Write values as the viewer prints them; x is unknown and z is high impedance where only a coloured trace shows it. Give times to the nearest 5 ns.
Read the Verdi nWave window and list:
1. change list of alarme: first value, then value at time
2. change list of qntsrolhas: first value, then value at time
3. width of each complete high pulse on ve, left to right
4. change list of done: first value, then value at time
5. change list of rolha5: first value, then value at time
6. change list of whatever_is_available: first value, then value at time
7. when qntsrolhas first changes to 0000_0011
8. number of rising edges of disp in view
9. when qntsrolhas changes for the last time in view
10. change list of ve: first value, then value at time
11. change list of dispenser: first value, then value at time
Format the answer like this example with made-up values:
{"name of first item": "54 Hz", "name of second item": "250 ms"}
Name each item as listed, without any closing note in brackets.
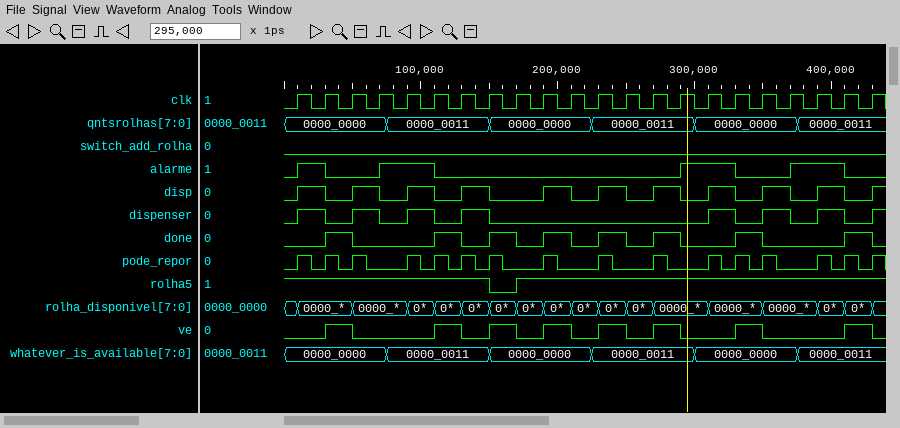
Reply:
{"change list of alarme: first value, then value at time": "0, 1 at 10 ns, 0 at 30 ns, 1 at 70 ns, 0 at 110 ns, 1 at 290 ns, 0 at 330 ns, 1 at 370 ns, 0 at 410 ns", "change list of qntsrolhas: first value, then value at time": "0000_0000, 0000_0011 at 75 ns, 0000_0000 at 150 ns, 0000_0011 at 225 ns, 0000_0000 at 300 ns, 0000_0011 at 375 ns", "width of each complete high pulse on ve, left to right": "20 ns, 20 ns, 20 ns, 20 ns, 20 ns, 20 ns, 20 ns, 20 ns", "change list of done: first value, then value at time": "0, 1 at 30 ns, 0 at 50 ns, 1 at 110 ns, 0 at 130 ns, 1 at 150 ns, 0 at 170 ns, 1 at 190 ns, 0 at 210 ns, 1 at 230 ns, 0 at 250 ns, 1 at 270 ns, 0 at 290 ns, 1 at 330 ns, 0 at 350 ns, 1 at 410 ns, 0 at 430 ns", "change list of rolha5: first value, then value at time": "1, 0 at 150 ns, 1 at 170 ns", "change list of whatever_is_available: first value, then value at time": "0000_0000, 0000_0011 at 75 ns, 0000_0000 at 150 ns, 0000_0011 at 225 ns, 0000_0000 at 300 ns, 0000_0011 at 375 ns", "when qntsrolhas first changes to 0000_0011": "75 ns", "number of rising edges of disp in view": "11", "when qntsrolhas changes for the last time in view": "375 ns", "change list of ve: first value, then value at time": "0, 1 at 30 ns, 0 at 50 ns, 1 at 110 ns, 0 at 130 ns, 1 at 150 ns, 0 at 170 ns, 1 at 190 ns, 0 at 210 ns, 1 at 230 ns, 0 at 250 ns, 1 at 270 ns, 0 at 290 ns, 1 at 330 ns, 0 at 350 ns, 1 at 410 ns, 0 at 430 ns", "change list of dispenser: first value, then value at time": "0, 1 at 10 ns, 0 at 30 ns, 1 at 50 ns, 0 at 70 ns, 1 at 90 ns, 0 at 110 ns, 1 at 130 ns, 0 at 150 ns, 1 at 310 ns, 0 at 330 ns, 1 at 350 ns, 0 at 370 ns, 1 at 390 ns, 0 at 410 ns, 1 at 430 ns"}
